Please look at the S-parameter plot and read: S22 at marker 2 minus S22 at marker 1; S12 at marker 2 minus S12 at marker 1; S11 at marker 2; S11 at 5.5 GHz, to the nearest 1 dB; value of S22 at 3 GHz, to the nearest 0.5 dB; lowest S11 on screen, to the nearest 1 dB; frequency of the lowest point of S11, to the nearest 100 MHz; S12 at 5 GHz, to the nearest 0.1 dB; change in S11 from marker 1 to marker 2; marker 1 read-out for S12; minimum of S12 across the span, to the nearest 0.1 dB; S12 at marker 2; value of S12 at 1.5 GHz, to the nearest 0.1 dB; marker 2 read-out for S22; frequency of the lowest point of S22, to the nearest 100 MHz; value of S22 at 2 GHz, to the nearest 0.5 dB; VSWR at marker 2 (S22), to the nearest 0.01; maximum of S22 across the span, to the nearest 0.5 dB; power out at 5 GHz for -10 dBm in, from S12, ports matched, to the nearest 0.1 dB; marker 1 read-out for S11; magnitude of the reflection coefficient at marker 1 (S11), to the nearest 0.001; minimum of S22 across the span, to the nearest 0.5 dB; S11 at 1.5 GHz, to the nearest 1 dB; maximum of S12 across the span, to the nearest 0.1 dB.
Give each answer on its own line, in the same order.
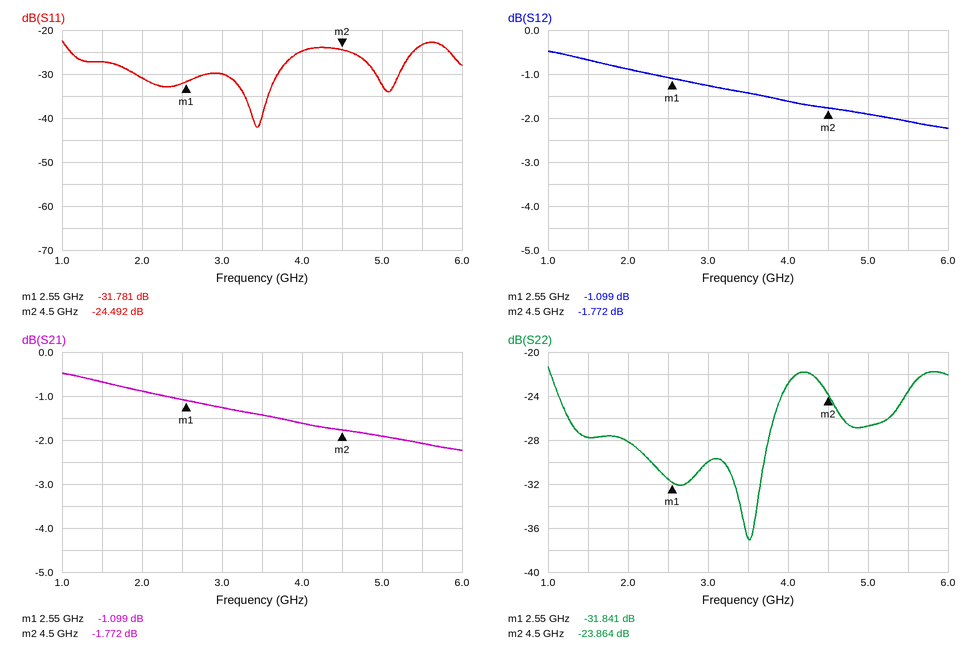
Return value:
7.977 dB
-0.673 dB
-24.492 dB
-23 dB
-30.0 dB
-42 dB
3.4 GHz
-1.9 dB
7.289 dB
-1.099 dB
-2.2 dB
-1.772 dB
-0.7 dB
-23.864 dB
3.5 GHz
-28.0 dB
1.14
-21.5 dB
-11.9 dBm
-31.781 dB
0.026
-37.0 dB
-27 dB
-0.5 dB
